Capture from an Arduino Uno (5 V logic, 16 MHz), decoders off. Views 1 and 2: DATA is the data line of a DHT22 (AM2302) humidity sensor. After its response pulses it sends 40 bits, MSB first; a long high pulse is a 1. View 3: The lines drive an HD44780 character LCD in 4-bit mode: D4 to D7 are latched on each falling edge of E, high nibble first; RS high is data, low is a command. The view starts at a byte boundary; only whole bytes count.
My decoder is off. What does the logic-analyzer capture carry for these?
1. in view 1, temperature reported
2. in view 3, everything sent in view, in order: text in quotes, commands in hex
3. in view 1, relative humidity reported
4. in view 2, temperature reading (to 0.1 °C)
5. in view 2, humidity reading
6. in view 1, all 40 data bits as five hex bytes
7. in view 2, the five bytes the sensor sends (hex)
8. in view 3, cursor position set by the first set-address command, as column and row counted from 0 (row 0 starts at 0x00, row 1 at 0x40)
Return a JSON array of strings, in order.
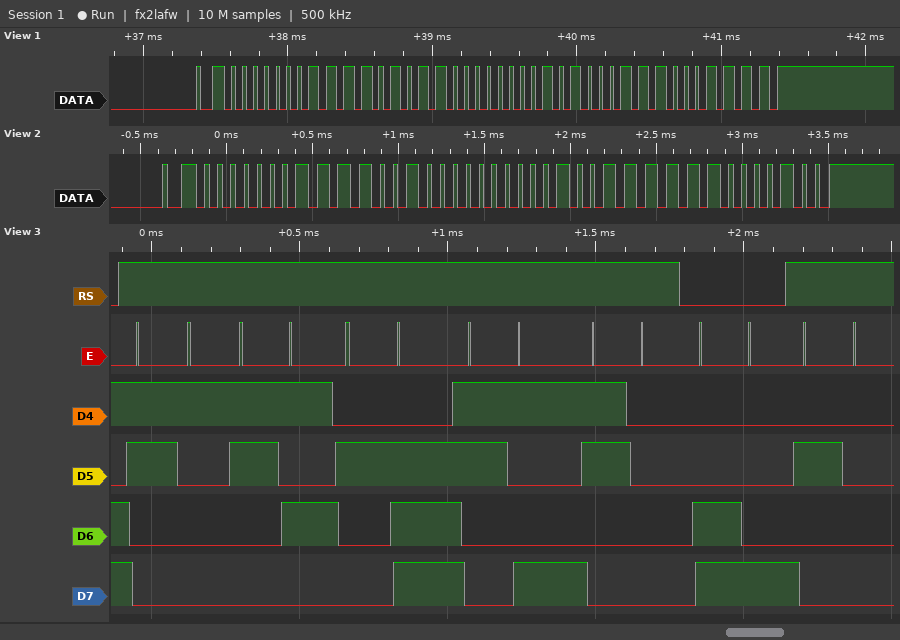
["16.3 °C", "\"15.90\" 0xC8 \" \"", "49.1 %", "15.9 °C", "48.4 %", "01 EB 00 A3 8F", "01 E4 00 9F 84", "column 8, row 1"]
